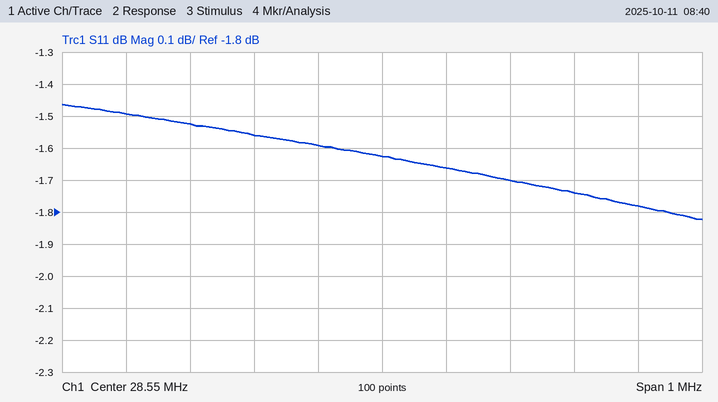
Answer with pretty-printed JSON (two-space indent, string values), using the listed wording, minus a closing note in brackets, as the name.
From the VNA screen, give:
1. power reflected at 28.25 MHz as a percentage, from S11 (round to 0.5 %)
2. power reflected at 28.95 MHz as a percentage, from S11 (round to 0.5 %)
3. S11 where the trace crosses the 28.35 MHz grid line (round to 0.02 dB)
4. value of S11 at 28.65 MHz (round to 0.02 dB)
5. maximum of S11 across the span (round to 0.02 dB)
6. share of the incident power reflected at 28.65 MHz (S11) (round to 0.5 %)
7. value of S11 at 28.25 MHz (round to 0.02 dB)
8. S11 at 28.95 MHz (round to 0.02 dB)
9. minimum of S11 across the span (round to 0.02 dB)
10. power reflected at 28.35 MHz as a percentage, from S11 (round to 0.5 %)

{
  "power reflected at 28.25 MHz as a percentage, from S11": "70.5 %",
  "power reflected at 28.95 MHz as a percentage, from S11": "66.5 %",
  "S11 where the trace crosses the 28.35 MHz grid line": "-1.56 dB",
  "value of S11 at 28.65 MHz": "-1.66 dB",
  "maximum of S11 across the span": "-1.46 dB",
  "share of the incident power reflected at 28.65 MHz (S11)": "68.0 %",
  "value of S11 at 28.25 MHz": "-1.52 dB",
  "S11 at 28.95 MHz": "-1.78 dB",
  "minimum of S11 across the span": "-1.82 dB",
  "power reflected at 28.35 MHz as a percentage, from S11": "70.0 %"
}
